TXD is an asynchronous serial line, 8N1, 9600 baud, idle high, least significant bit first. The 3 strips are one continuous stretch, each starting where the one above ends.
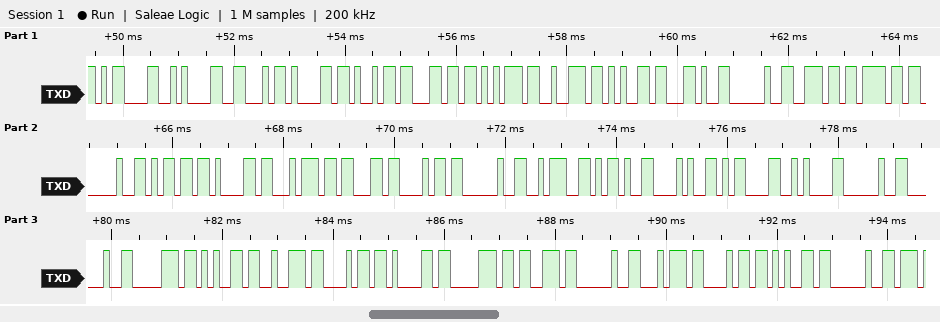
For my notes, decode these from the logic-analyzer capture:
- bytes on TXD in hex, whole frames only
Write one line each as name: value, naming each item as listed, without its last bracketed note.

bytes on TXD in hex, whole frames only: 0D 0A 46 61 69 6C 75 72 65 2C 20 6E 6F 20 6D 61 74 63 68 20 3A 2D 28 0D 0A 20 20 70 65 72 68 61 70 73 20 74 68 65 20
